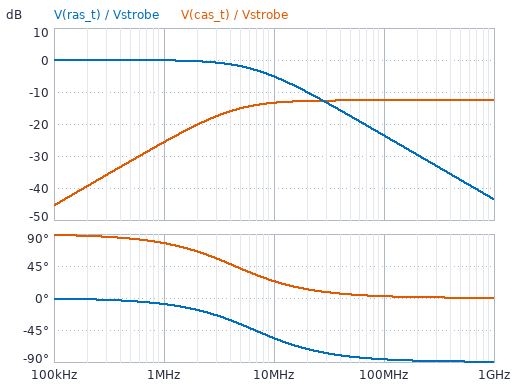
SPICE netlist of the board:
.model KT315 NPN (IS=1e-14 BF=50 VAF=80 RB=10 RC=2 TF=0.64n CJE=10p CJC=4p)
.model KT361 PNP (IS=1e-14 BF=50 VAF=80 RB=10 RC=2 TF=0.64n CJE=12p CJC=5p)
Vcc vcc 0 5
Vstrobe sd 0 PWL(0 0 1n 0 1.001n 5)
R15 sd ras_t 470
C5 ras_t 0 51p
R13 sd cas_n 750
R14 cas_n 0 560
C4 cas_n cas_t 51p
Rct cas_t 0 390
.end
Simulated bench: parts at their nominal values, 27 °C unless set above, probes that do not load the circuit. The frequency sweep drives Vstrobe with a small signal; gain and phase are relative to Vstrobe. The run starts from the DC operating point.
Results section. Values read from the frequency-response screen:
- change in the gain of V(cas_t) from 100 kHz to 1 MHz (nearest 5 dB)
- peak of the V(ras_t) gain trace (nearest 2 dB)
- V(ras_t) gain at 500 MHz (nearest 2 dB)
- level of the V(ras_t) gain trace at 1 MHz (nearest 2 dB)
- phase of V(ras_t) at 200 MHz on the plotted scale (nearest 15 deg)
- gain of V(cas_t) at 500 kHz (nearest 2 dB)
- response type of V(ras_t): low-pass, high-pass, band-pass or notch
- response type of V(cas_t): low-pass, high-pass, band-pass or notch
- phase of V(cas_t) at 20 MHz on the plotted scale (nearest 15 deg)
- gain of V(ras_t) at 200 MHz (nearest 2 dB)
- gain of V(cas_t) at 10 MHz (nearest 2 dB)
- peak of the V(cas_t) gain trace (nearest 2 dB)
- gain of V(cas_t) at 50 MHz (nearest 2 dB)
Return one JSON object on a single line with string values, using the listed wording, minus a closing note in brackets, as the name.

{"change in the gain of V(cas_t) from 100 kHz to 1 MHz": "20 dB", "peak of the V(ras_t) gain trace": "0 dB", "V(ras_t) gain at 500 MHz": "-38 dB", "level of the V(ras_t) gain trace at 1 MHz": "0 dB", "phase of V(ras_t) at 200 MHz on the plotted scale": "-90 deg", "gain of V(cas_t) at 500 kHz": "-32 dB", "response type of V(ras_t): low-pass, high-pass, band-pass or notch": "low-pass", "response type of V(cas_t): low-pass, high-pass, band-pass or notch": "high-pass", "phase of V(cas_t) at 20 MHz on the plotted scale": "15 deg", "gain of V(ras_t) at 200 MHz": "-30 dB", "gain of V(cas_t) at 10 MHz": "-14 dB", "peak of the V(cas_t) gain trace": "-12 dB", "gain of V(cas_t) at 50 MHz": "-12 dB"}
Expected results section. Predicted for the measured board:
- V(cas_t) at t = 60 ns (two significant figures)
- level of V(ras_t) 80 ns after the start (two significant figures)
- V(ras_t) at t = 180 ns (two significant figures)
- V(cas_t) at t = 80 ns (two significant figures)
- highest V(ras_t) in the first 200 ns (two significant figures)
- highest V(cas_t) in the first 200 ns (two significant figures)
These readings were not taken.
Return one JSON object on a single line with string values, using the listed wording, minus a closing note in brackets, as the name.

{"V(cas_t) at t = 60 ns": "230 mV", "level of V(ras_t) 80 ns after the start": "4.8 V", "V(ras_t) at t = 180 ns": "5.0 V", "V(cas_t) at t = 80 ns": "130 mV", "highest V(ras_t) in the first 200 ns": "5.0 V", "highest V(cas_t) in the first 200 ns": "1.2 V"}
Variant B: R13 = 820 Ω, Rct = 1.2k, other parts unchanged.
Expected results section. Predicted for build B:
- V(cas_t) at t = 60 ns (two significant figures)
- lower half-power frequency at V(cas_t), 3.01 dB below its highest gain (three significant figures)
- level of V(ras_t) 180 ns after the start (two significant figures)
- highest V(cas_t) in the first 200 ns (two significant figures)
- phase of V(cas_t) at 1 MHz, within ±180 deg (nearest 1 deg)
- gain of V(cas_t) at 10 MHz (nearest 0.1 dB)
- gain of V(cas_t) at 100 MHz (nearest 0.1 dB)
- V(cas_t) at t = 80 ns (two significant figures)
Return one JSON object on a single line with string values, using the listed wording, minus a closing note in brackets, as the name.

{"V(cas_t) at t = 60 ns": "750 mV", "lower half-power frequency at V(cas_t), 3.01 dB below its highest gain": "2.04 MHz", "level of V(ras_t) 180 ns after the start": "5.0 V", "highest V(cas_t) in the first 200 ns": "1.6 V", "phase of V(cas_t) at 1 MHz, within ±180 deg": "64 deg", "gain of V(cas_t) at 10 MHz": "-10.1 dB", "gain of V(cas_t) at 100 MHz": "-10.0 dB", "V(cas_t) at t = 80 ns": "580 mV"}
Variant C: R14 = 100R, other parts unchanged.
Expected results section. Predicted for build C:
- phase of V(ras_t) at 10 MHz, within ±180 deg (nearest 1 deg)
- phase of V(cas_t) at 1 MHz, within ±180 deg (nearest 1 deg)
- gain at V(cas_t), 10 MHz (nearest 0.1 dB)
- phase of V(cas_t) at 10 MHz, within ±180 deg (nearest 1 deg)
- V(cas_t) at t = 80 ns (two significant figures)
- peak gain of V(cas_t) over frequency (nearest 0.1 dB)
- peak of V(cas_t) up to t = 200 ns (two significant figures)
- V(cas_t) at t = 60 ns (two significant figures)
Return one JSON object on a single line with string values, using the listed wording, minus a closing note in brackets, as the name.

{"phase of V(ras_t) at 10 MHz, within ±180 deg": "-56 deg", "phase of V(cas_t) at 1 MHz, within ±180 deg": "81 deg", "gain at V(cas_t), 10 MHz": "-21.9 dB", "phase of V(cas_t) at 10 MHz, within ±180 deg": "33 deg", "V(cas_t) at t = 80 ns": "19 mV", "peak gain of V(cas_t) over frequency": "-20.4 dB", "peak of V(cas_t) up to t = 200 ns": "480 mV", "V(cas_t) at t = 60 ns": "43 mV"}
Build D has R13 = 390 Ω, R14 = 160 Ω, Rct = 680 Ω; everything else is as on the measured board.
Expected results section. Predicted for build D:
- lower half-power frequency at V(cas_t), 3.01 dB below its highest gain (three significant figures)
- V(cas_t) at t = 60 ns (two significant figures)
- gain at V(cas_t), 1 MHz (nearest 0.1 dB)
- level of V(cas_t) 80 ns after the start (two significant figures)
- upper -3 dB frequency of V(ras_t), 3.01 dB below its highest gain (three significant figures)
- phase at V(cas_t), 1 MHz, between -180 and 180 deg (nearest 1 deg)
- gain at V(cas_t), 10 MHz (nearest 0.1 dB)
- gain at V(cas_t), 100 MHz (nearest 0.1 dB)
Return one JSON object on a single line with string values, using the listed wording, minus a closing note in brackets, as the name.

{"lower half-power frequency at V(cas_t), 3.01 dB below its highest gain": "3.93 MHz", "V(cas_t) at t = 60 ns": "290 mV", "gain at V(cas_t), 1 MHz": "-24.2 dB", "level of V(cas_t) 80 ns after the start": "180 mV", "upper -3 dB frequency of V(ras_t), 3.01 dB below its highest gain": "6.64 MHz", "phase at V(cas_t), 1 MHz, between -180 and 180 deg": "76 deg", "gain at V(cas_t), 10 MHz": "-12.7 dB", "gain at V(cas_t), 100 MHz": "-12.1 dB"}
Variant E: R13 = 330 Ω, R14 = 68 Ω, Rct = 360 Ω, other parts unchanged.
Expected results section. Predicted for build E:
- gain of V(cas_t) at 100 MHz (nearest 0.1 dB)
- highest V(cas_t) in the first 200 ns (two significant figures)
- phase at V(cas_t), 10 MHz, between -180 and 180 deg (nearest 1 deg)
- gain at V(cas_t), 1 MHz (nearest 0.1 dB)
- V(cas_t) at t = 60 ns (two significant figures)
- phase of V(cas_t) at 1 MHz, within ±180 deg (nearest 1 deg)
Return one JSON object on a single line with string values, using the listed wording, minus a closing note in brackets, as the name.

{"gain of V(cas_t) at 100 MHz": "-16.6 dB", "highest V(cas_t) in the first 200 ns": "740 mV", "phase at V(cas_t), 10 MHz, between -180 and 180 deg": "37 deg", "gain at V(cas_t), 1 MHz": "-34.2 dB", "V(cas_t) at t = 60 ns": "46 mV", "phase of V(cas_t) at 1 MHz, within ±180 deg": "82 deg"}
